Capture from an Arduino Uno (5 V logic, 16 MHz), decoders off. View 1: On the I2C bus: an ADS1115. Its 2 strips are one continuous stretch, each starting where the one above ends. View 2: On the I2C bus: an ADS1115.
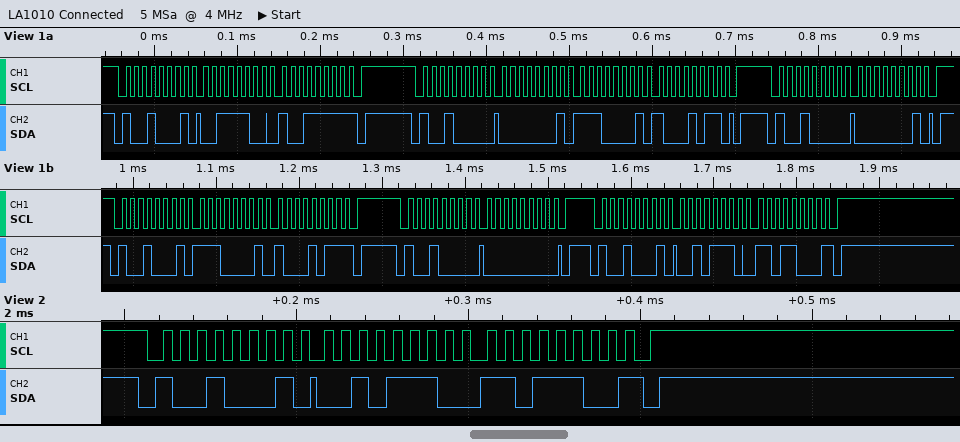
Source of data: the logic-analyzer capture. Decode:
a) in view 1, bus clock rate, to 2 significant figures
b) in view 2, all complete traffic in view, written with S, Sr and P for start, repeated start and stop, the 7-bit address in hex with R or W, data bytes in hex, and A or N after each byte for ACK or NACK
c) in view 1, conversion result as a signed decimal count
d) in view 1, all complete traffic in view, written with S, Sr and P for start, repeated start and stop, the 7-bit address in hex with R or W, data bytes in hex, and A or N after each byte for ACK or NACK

100 kHz
S 48R A 2E A DC N P
11992
S 48R A 3C A 9F N P S 48W A 01 A E1 A 8B A P S 48W A 01 A P S 48R A E1 A 8B N P S 48W A 00 A P S 48R A 2E A D8 N P
